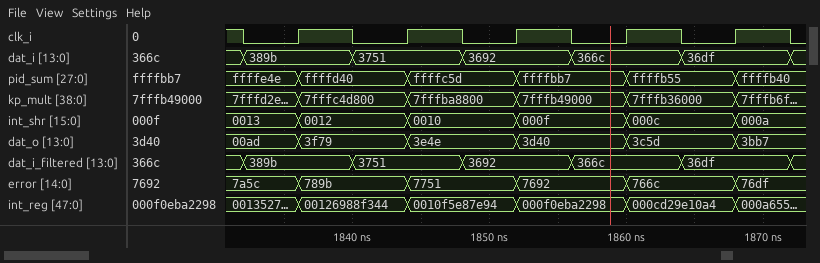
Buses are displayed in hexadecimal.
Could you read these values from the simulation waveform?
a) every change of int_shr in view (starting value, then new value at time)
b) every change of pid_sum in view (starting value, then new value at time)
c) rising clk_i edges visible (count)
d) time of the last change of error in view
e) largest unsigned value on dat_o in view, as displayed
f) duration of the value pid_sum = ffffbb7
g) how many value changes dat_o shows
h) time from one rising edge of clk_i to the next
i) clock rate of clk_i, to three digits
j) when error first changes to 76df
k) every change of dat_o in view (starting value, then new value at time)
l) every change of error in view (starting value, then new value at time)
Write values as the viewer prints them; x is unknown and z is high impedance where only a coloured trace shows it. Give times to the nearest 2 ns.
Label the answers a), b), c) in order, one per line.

a) 0013, 0012 at 1836 ns, 0010 at 1844 ns, 000f at 1852 ns, 000c at 1860 ns, 000a at 1868 ns
b) ffffe4e, ffffd40 at 1836 ns, ffffc5d at 1844 ns, ffffbb7 at 1852 ns, ffffb55 at 1860 ns, ffffb40 at 1868 ns
c) 5
d) 1868 ns
e) 3f79
f) 8 ns
g) 5
h) 8 ns
i) 125 MHz
j) 1868 ns
k) 00ad, 3f79 at 1836 ns, 3e4e at 1844 ns, 3d40 at 1852 ns, 3c5d at 1860 ns, 3bb7 at 1868 ns
l) 7a5c, 789b at 1836 ns, 7751 at 1844 ns, 7692 at 1852 ns, 766c at 1860 ns, 76df at 1868 ns
